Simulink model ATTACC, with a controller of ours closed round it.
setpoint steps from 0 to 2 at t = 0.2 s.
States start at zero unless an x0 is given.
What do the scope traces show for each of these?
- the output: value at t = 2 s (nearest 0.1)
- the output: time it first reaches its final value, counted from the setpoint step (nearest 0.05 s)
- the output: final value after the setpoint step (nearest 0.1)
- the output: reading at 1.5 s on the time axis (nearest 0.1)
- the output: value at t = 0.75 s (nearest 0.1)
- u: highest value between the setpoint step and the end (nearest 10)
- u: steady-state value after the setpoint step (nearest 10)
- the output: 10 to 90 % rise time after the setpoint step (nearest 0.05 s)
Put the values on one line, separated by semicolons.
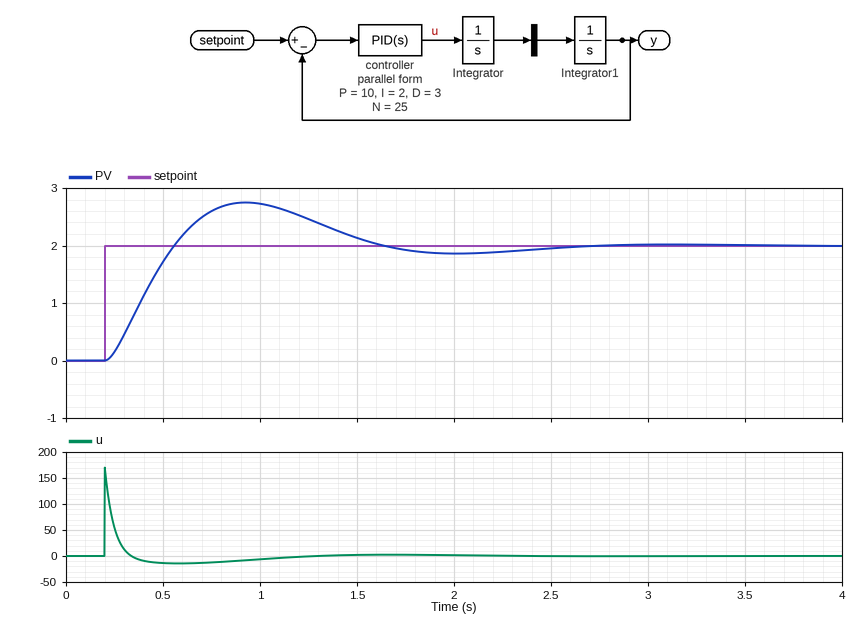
1.9; 0.35 s; 2.0; 2.1; 2.6; 170; 0; 0.25 s
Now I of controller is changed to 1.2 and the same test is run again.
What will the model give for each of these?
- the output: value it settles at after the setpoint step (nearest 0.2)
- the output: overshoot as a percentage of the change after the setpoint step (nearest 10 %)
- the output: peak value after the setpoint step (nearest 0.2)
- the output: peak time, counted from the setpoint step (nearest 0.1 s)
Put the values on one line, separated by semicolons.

2.0; 40 %; 2.8; 0.7 s
